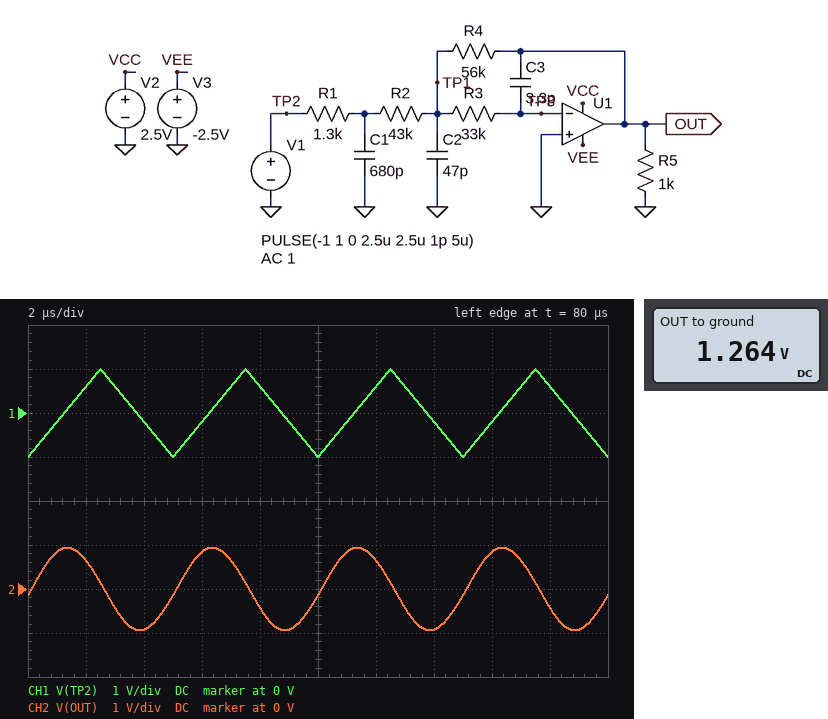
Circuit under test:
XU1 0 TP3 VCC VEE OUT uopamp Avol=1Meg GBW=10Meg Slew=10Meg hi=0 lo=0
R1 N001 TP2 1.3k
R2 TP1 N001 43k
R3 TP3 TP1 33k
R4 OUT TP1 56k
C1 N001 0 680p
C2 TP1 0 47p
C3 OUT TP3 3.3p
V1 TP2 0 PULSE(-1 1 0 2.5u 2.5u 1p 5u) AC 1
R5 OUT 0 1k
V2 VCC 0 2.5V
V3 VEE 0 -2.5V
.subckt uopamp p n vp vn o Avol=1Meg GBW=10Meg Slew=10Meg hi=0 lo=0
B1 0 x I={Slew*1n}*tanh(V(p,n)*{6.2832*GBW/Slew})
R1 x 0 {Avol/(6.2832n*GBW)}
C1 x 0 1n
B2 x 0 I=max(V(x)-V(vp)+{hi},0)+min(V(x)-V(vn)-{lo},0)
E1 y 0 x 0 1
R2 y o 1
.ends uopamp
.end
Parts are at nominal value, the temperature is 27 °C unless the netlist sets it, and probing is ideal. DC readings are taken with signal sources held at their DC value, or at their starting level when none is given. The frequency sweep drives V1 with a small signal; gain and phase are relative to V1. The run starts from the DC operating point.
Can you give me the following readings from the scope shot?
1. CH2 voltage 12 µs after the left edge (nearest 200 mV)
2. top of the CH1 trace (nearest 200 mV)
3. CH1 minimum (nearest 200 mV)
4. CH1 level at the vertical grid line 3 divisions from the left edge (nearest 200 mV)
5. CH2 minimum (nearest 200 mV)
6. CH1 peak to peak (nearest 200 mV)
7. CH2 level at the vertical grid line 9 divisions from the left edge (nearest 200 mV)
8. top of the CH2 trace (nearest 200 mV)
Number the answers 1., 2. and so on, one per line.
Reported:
1. 600 mV
2. 1.0 V
3. -1.0 V
4. -200 mV
5. -1.0 V
6. 2.0 V
7. -400 mV
8. 1.0 V
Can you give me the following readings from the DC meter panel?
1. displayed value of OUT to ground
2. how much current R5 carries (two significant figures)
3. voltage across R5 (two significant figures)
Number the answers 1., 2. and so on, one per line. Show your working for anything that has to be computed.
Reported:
1. 1.264 V
2. (1.264 V) / 1 kΩ = 1.3 mA
3. 1.264 V = 1.3 V
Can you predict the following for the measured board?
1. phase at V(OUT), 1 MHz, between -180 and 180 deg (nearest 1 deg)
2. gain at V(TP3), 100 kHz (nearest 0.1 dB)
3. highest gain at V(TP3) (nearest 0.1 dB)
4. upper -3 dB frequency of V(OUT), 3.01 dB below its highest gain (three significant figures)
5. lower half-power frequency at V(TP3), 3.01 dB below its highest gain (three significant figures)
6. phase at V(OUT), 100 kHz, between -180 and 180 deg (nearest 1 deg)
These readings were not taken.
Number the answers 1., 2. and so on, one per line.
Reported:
1. -71 deg
2. -38.3 dB
3. -31.9 dB
4. 275 kHz
5. 151 kHz
6. 133 deg
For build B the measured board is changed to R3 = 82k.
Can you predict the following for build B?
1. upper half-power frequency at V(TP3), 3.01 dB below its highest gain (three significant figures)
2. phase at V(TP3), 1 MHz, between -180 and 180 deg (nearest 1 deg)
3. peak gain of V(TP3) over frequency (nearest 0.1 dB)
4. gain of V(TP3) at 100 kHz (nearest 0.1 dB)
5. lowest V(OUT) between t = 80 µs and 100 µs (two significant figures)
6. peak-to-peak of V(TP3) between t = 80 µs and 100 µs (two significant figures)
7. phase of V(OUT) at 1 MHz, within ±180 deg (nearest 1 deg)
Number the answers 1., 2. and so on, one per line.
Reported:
1. 243 kHz
2. -165 deg
3. -35.0 dB
4. -37.8 dB
5. -660 mV
6. 27 mV
7. -75 deg
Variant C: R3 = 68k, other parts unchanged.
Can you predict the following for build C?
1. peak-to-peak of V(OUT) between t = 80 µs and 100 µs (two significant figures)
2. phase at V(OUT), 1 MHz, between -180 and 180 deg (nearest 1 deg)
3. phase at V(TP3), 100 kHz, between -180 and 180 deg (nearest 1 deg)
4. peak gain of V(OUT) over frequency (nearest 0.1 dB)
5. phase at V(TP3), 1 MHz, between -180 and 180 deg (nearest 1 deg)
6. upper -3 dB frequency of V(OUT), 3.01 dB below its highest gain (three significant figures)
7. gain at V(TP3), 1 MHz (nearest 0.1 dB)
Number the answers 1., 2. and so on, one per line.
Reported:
1. 1.5 V
2. -74 deg
3. 30 deg
4. 2.1 dB
5. -164 deg
6. 207 kHz
7. -60.5 dB
